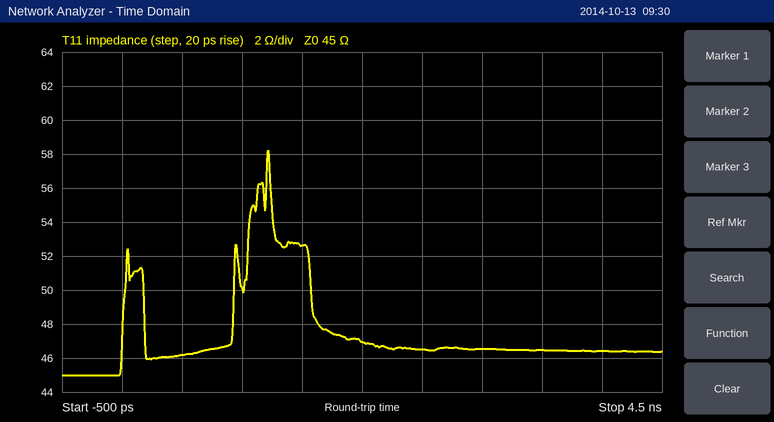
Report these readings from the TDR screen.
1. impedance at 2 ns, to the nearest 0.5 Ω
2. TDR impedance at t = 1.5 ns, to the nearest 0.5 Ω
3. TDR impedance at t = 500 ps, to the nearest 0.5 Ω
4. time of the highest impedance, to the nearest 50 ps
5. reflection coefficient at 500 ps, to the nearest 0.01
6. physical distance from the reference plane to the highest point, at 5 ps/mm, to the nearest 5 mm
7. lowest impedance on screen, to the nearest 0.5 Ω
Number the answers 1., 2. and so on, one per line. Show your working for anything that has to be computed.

1. 47.0 Ω
2. 52.5 Ω
3. 46.0 Ω
4. 1.20 ns
5. (46 − 45)/(46 + 45) ≈ +0.01
6. 1.20 ns / 2 / 5 ps/mm ≈ 120 mm
7. 45.0 Ω
